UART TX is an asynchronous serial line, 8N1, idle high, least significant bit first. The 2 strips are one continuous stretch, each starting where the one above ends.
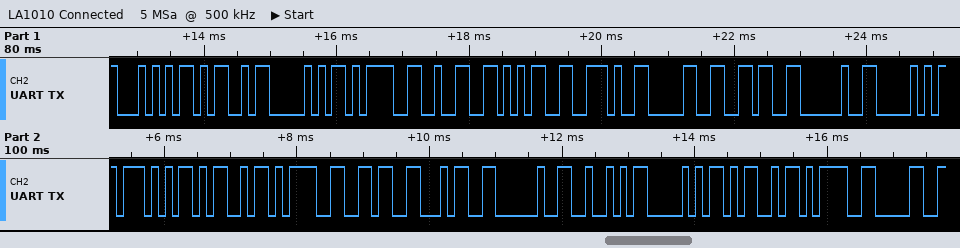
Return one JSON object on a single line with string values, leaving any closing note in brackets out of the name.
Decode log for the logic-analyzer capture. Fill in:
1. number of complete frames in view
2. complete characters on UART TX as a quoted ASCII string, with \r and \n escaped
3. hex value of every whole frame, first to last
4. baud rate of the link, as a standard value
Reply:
{"number of complete frames in view": "22", "complete characters on UART TX as a quoted ASCII string, with \\r and \\n escaped": "\"TMP=25.06 PWM=64 RPM=0\"", "hex value of every whole frame, first to last": "54 4D 50 3D 32 35 2E 30 36 20 50 57 4D 3D 36 34 20 52 50 4D 3D 30", "baud rate of the link, as a standard value": "9600 baud"}
